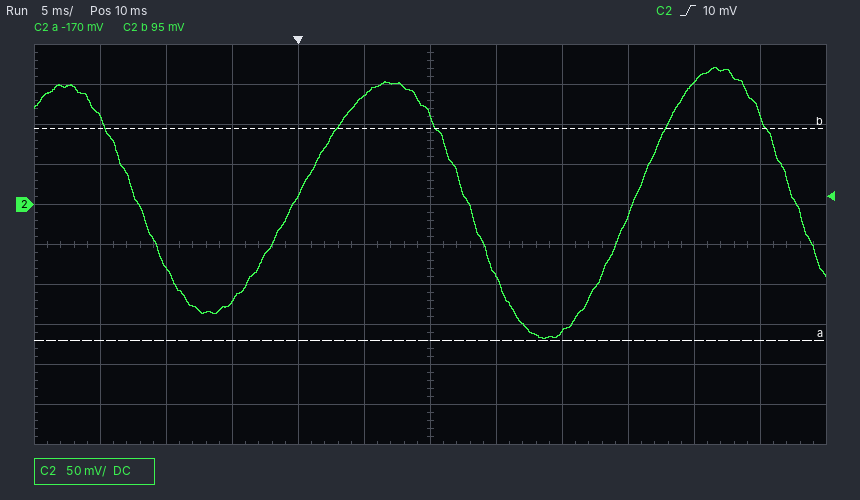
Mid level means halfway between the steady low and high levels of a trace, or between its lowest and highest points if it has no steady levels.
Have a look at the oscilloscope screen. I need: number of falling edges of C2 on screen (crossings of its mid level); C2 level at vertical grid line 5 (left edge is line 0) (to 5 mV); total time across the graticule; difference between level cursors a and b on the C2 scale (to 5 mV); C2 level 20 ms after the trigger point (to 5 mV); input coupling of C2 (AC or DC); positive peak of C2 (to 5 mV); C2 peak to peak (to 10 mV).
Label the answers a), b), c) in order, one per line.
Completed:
a) 3
b) 135 mV
c) 60 ms
d) 265 mV
e) -160 mV
f) DC
g) 170 mV
h) 340 mV
